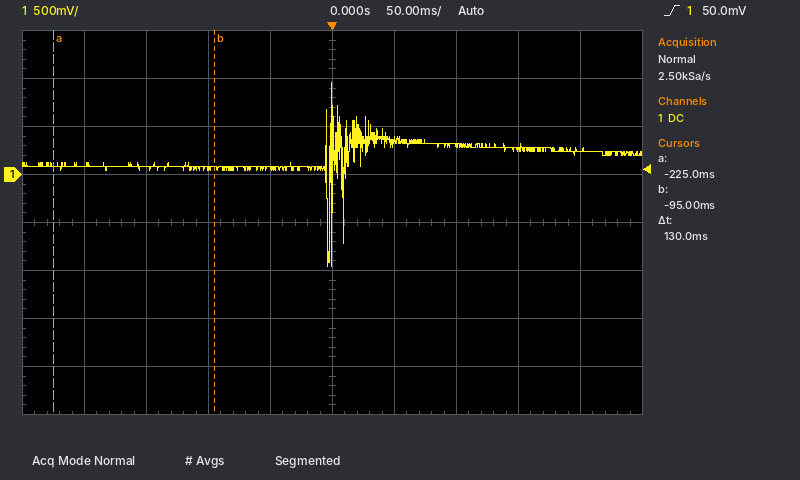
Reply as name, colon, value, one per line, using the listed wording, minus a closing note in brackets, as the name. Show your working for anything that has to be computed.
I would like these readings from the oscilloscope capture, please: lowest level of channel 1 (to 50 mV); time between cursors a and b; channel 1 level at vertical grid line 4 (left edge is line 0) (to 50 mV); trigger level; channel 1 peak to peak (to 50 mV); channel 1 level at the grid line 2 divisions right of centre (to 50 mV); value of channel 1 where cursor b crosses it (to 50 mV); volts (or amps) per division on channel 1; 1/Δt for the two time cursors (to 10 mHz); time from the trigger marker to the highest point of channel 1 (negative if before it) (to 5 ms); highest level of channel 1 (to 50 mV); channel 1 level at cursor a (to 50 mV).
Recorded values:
lowest level of channel 1: -950 mV
time between cursors a and b: 130 ms
channel 1 level at vertical grid line 4 (left edge is line 0): 50 mV
trigger level: 50.0 mV
channel 1 peak to peak: 950 mV − (-950 mV) = 1.90 V
channel 1 level at the grid line 2 divisions right of centre: 300 mV
value of channel 1 where cursor b crosses it: 50 mV
volts (or amps) per division on channel 1: 500 mV
1/Δt for the two time cursors: 1 / 130 ms ≈ 7.69 Hz
time from the trigger marker to the highest point of channel 1 (negative if before it): 0 ms
highest level of channel 1: 950 mV
channel 1 level at cursor a: 100 mV
